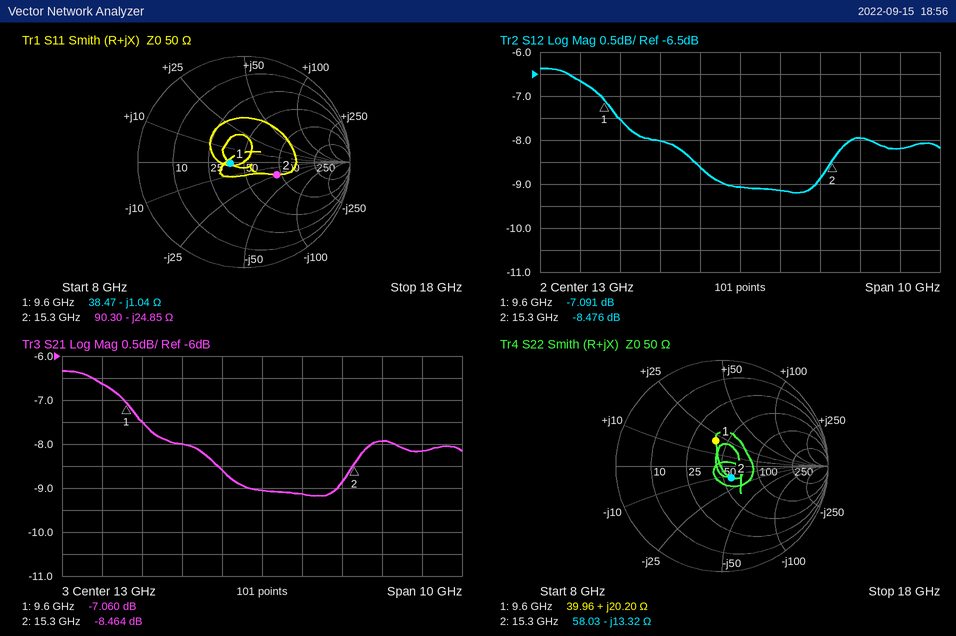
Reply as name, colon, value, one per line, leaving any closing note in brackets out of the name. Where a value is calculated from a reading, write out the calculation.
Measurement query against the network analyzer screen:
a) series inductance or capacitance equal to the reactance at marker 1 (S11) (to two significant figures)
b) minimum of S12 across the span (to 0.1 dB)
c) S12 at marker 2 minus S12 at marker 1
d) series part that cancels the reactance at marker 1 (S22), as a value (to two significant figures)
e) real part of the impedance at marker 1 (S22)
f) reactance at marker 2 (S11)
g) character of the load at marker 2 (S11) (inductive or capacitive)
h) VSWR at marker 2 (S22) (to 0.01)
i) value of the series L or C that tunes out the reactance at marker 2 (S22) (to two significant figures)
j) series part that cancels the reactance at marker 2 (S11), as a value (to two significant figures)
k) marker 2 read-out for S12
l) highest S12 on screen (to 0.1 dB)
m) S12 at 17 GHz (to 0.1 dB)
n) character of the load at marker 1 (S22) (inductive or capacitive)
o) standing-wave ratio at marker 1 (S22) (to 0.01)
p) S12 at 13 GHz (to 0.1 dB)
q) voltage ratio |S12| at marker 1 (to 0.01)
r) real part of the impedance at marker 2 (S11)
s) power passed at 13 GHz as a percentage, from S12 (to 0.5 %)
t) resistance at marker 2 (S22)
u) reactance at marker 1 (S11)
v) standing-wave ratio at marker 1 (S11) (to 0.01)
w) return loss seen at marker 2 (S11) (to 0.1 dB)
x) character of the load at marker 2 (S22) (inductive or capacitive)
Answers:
series inductance or capacitance equal to the reactance at marker 1 (S11): C = 1/(2π × 9.6 GHz × 1.04 Ω) ≈ 16 pF
minimum of S12 across the span: -9.2 dB
S12 at marker 2 minus S12 at marker 1: -8.476 − (-7.091) = -1.385 dB
series part that cancels the reactance at marker 1 (S22), as a value: C = 1/(2π × 9.6 GHz × 20.2 Ω) ≈ 821 fF, so 820 fF to two significant figures
real part of the impedance at marker 1: 39.96 Ω
reactance at marker 2: -24.85 Ω
character of the load at marker 2 (S11): capacitive
VSWR at marker 2 (S22): 1.33
value of the series L or C that tunes out the reactance at marker 2 (S22): L = 13.32 Ω/(2π × 15.3 GHz) ≈ 139 pH, so 140 pH to two significant figures
series part that cancels the reactance at marker 2 (S11), as a value: L = 24.85 Ω/(2π × 15.3 GHz) ≈ 258 pH, so 260 pH to two significant figures
marker 2 read-out for S12: -8.476 dB
highest S12 on screen: -6.4 dB
S12 at 17 GHz: -8.2 dB
character of the load at marker 1 (S22): inductive
standing-wave ratio at marker 1 (S22): 1.65
S12 at 13 GHz: -9.1 dB
voltage ratio |S12| at marker 1: 10^(-7.091/20) ≈ 0.44
real part of the impedance at marker 2: 90.30 Ω
power passed at 13 GHz as a percentage, from S12: 10^(-9.1/10) ≈ 12.3 %, so 12.5 % to the nearest 0.5 %
resistance at marker 2: 58.03 Ω
reactance at marker 1: -1.04 Ω
standing-wave ratio at marker 1 (S11): 1.30
return loss seen at marker 2 (S11): 9.6 dB
character of the load at marker 2 (S22): capacitive
